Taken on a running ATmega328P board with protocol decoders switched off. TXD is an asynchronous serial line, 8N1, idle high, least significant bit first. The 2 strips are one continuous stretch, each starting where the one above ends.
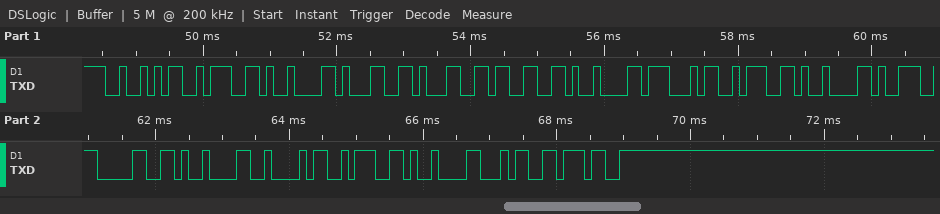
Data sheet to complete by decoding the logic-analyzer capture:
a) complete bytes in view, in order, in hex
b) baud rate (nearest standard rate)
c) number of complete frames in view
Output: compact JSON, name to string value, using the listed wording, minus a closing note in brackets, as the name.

{"complete bytes in view, in order, in hex": "52 3A 09 31 31 33 09 47 3A 09 39 30 09 42 3A 09 34 37", "baud rate": "9600 baud", "number of complete frames in view": "18"}
